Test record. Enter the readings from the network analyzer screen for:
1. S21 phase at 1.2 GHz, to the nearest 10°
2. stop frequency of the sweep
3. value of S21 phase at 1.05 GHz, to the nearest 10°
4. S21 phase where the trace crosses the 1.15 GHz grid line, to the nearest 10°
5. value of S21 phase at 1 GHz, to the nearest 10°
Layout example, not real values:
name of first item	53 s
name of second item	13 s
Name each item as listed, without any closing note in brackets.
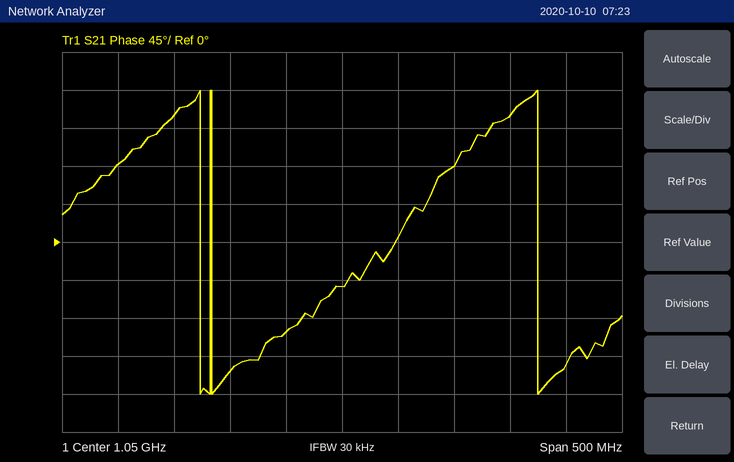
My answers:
S21 phase at 1.2 GHz, to the nearest 10°	150°
stop frequency of the sweep	1.3 GHz
value of S21 phase at 1.05 GHz, to the nearest 10°	-50°
S21 phase where the trace crosses the 1.15 GHz grid line, to the nearest 10°	90°
value of S21 phase at 1 GHz, to the nearest 10°	-110°
